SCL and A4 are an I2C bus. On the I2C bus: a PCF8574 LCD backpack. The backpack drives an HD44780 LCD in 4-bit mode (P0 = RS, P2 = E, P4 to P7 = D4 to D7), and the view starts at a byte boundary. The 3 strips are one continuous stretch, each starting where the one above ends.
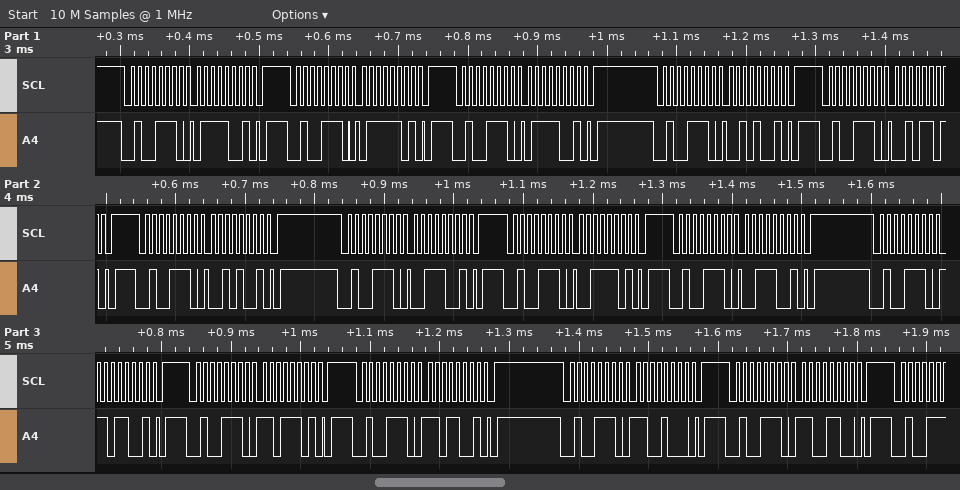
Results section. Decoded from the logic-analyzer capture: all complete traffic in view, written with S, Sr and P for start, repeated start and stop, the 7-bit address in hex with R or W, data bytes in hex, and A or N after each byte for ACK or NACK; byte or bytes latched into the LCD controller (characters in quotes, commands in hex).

S 27W A 79 A P S 27W A 7D A P S 27W A 79 A P S 27W A 29 A P S 27W A 2D A P S 27W A 29 A P S 27W A 39 A P S 27W A 3D A P S 27W A 39 A P S 27W A D9 A P S 27W A DD A P S 27W A D9 A P S 27W A C8 A P S 27W A CC A P
'r' '='
